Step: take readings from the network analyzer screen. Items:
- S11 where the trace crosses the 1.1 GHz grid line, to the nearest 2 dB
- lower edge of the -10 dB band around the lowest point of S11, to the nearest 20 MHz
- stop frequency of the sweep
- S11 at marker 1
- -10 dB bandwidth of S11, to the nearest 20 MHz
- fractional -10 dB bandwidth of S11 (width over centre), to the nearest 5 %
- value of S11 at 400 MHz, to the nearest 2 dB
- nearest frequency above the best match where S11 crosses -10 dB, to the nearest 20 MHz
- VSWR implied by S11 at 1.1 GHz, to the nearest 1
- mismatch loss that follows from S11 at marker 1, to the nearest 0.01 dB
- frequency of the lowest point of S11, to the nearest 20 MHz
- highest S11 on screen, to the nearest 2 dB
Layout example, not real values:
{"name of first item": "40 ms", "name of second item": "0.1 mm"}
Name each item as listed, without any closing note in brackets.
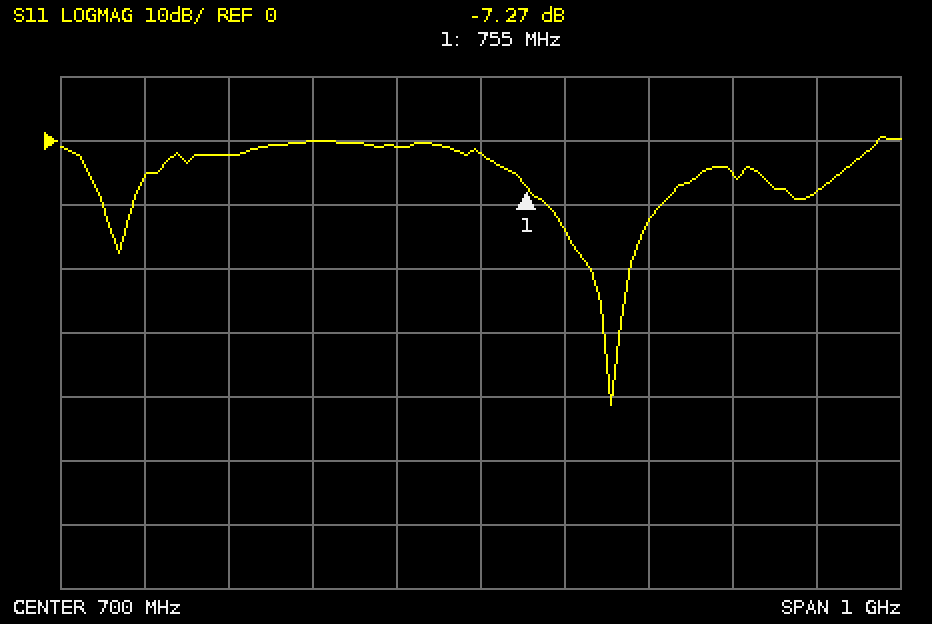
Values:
{"S11 where the trace crosses the 1.1 GHz grid line, to the nearest 2 dB": "-8 dB", "lower edge of the -10 dB band around the lowest point of S11, to the nearest 20 MHz": "780 MHz", "stop frequency of the sweep": "1.2 GHz", "S11 at marker 1": "-7.27 dB", "-10 dB bandwidth of S11, to the nearest 20 MHz": "140 MHz", "fractional -10 dB bandwidth of S11 (width over centre), to the nearest 5 %": "15 %", "value of S11 at 400 MHz, to the nearest 2 dB": "-2 dB", "nearest frequency above the best match where S11 crosses -10 dB, to the nearest 20 MHz": "920 MHz", "VSWR implied by S11 at 1.1 GHz, to the nearest 1": "2", "mismatch loss that follows from S11 at marker 1, to the nearest 0.01 dB": "0.90 dB", "frequency of the lowest point of S11, to the nearest 20 MHz": "860 MHz", "highest S11 on screen, to the nearest 2 dB": "0 dB"}
